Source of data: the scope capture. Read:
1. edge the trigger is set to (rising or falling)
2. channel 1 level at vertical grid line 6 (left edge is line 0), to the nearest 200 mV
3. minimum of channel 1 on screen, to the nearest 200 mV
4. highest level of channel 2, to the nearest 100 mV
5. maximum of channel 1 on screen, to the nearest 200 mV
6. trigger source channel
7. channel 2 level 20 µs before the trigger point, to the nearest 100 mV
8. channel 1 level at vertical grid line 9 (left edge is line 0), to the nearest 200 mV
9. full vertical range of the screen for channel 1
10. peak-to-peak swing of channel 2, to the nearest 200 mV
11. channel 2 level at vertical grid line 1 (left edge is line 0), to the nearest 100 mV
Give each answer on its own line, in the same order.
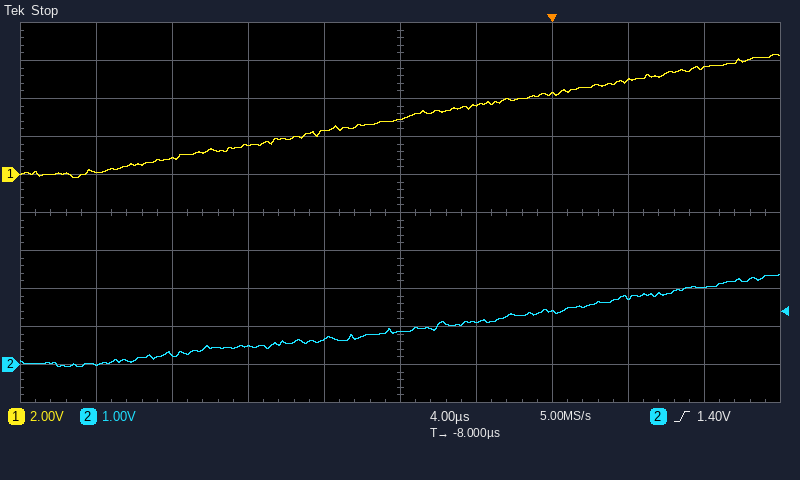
rising
3.6 V
-200 mV
2.4 V
6.4 V
channel 2
300 mV
5.6 V
20 V
2.4 V
0.0 V
